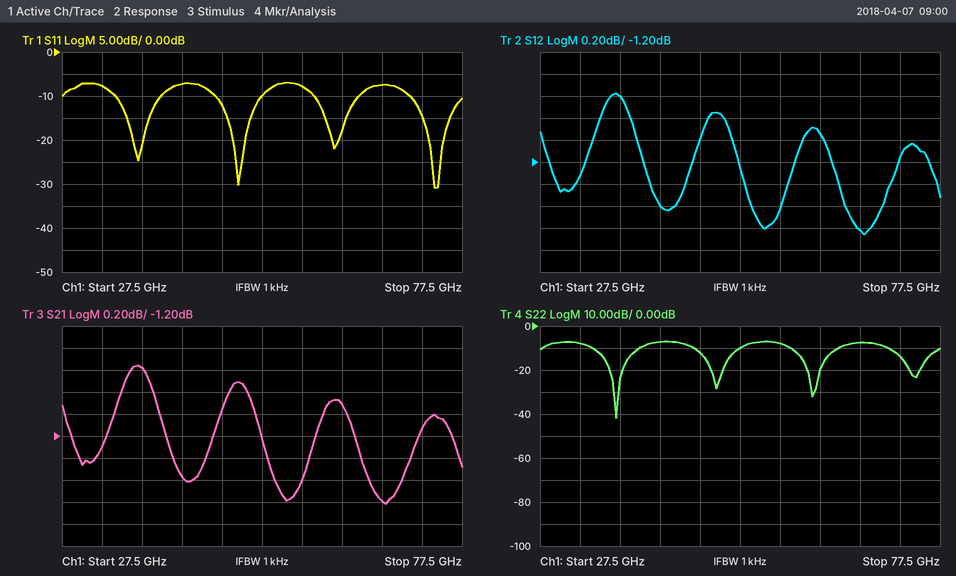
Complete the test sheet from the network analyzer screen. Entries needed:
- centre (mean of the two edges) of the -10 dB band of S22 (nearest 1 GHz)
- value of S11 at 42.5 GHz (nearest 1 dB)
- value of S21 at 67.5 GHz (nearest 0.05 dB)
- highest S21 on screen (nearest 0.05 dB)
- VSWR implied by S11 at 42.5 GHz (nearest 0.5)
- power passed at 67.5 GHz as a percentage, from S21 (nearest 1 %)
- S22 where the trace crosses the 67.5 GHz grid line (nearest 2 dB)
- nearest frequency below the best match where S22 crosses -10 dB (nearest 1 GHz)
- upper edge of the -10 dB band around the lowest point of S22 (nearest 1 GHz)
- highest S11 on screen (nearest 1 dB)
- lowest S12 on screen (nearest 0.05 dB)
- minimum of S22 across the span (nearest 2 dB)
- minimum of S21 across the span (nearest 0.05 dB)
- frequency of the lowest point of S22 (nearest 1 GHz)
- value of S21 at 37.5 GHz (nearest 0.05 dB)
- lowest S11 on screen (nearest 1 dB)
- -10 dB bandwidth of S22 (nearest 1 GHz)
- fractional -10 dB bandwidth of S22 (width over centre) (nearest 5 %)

37 GHz
-7 dB
-1.80 dB
-0.55 dB
2.5
66 %
-8 dB
34 GHz
40 GHz
-7 dB
-1.85 dB
-42 dB
-1.80 dB
37 GHz
-0.60 dB
-31 dB
6 GHz
15 %
